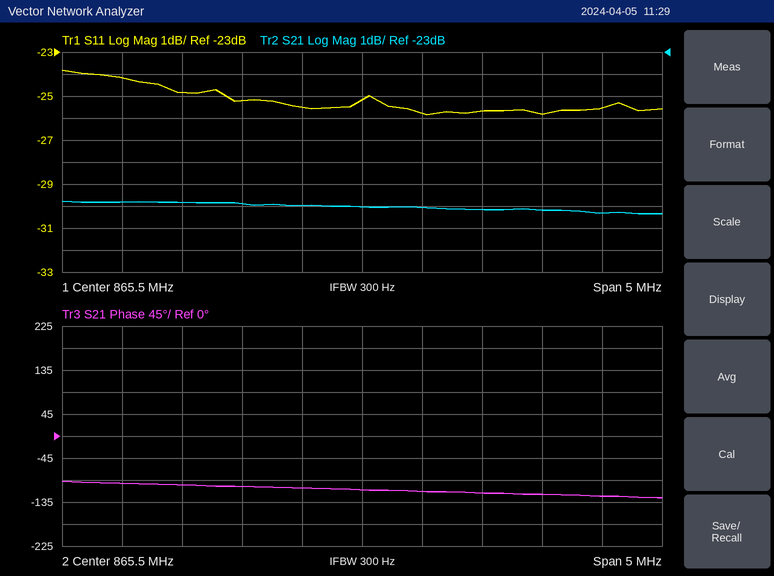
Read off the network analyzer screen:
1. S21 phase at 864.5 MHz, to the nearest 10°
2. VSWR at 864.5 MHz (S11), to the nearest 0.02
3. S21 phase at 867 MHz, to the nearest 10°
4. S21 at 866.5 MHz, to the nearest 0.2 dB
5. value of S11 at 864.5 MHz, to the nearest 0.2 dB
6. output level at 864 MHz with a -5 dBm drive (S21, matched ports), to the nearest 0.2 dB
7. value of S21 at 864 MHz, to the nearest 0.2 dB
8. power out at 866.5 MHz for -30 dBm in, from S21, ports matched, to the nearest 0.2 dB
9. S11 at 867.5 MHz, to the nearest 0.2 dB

-100°
1.12
-120°
-30.2 dB
-25.2 dB
-34.8 dBm
-29.8 dB
-60.2 dBm
-25.6 dB
